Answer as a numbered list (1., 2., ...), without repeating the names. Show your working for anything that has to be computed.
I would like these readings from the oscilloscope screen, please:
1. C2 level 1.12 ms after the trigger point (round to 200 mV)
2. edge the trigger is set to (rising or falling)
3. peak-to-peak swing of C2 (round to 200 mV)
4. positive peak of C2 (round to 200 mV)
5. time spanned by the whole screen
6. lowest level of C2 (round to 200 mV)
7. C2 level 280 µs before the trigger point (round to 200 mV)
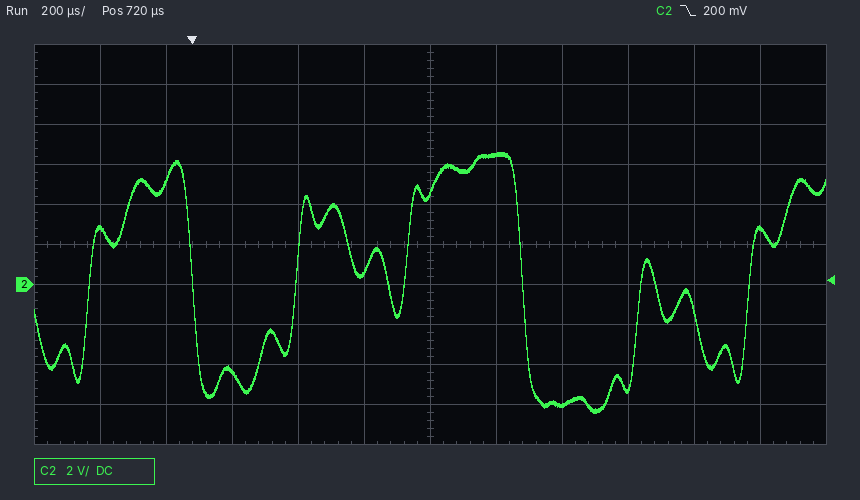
1. -6.0 V
2. falling
3. 6.6 V − (-6.4 V) = 13.0 V
4. 6.6 V
5. 2.4 ms
6. -6.4 V
7. 2.8 V
